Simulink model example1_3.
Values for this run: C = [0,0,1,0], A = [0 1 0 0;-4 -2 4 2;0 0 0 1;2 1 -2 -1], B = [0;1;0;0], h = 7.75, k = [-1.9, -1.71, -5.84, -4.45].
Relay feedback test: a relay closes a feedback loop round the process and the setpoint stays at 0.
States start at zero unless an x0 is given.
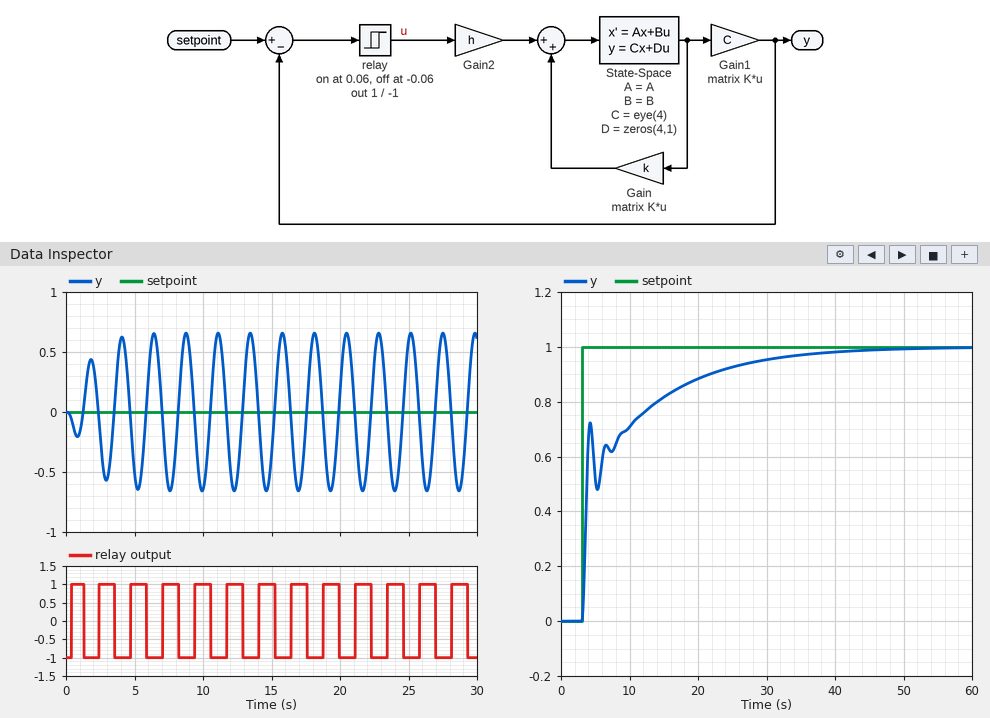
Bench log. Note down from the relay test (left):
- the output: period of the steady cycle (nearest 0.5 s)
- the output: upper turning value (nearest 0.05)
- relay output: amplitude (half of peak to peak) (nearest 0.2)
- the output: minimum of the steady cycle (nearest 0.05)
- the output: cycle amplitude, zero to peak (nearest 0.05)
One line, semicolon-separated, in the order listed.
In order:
2.5 s; 0.65; 1.0; -0.65; 0.65
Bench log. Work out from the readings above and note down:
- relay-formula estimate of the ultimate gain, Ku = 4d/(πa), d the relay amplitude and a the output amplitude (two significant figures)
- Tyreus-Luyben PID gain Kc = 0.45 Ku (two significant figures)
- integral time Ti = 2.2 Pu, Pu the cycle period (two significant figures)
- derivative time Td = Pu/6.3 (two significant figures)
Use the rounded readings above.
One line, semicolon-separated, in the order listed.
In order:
2.0; 0.90; 5.5 s; 0.40 s
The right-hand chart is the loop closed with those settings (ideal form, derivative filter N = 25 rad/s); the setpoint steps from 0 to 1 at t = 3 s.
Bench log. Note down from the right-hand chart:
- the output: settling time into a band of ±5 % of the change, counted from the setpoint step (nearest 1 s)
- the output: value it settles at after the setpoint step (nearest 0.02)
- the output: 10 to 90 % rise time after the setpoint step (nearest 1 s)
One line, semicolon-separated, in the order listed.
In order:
26 s; 1.00; 18 s
